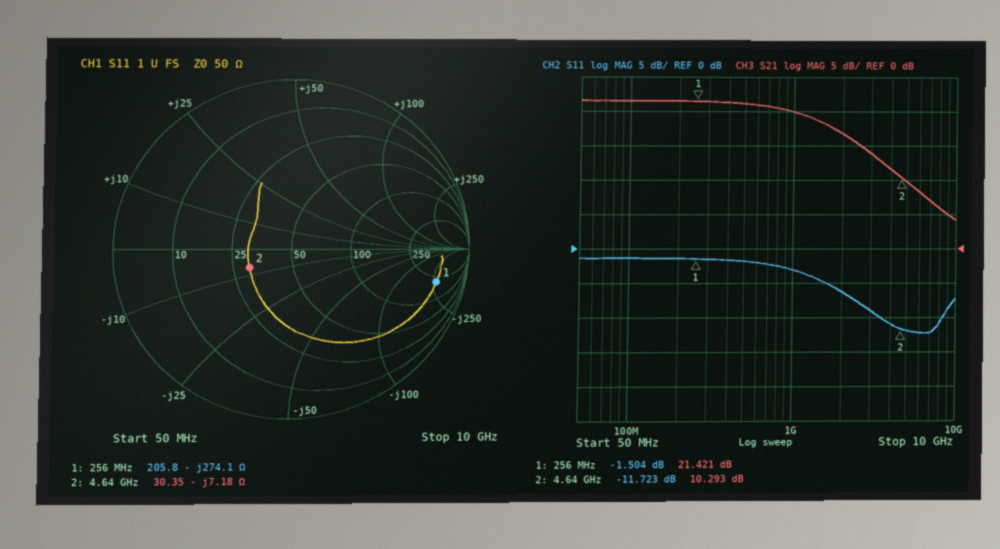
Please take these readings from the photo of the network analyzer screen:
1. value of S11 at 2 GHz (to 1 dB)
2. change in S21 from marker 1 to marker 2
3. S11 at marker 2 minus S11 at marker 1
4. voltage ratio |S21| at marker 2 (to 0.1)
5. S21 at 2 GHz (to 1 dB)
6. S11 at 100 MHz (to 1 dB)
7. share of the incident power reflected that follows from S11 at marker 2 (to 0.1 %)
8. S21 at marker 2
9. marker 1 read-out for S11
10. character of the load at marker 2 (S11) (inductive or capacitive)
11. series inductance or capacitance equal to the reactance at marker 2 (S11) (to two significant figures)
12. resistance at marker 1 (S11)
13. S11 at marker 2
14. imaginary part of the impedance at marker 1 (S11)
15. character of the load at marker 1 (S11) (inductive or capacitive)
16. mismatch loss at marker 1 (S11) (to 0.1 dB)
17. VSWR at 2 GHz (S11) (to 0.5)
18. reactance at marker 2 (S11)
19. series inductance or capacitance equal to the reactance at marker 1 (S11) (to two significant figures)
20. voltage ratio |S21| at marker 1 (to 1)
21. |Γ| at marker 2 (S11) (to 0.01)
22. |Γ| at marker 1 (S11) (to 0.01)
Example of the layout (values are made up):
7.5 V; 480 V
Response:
-6 dB; -11.128 dB; -10.219 dB; 3.3; 17 dB; -1 dB; 6.7 %; 10.293 dB; -1.504 dB; capacitive; 4.8 pF; 205.8 Ω; -11.723 dB; -274.1 Ω; capacitive; 5.3 dB; 3.0; -7.18 Ω; 2.3 pF; 12; 0.26; 0.84
